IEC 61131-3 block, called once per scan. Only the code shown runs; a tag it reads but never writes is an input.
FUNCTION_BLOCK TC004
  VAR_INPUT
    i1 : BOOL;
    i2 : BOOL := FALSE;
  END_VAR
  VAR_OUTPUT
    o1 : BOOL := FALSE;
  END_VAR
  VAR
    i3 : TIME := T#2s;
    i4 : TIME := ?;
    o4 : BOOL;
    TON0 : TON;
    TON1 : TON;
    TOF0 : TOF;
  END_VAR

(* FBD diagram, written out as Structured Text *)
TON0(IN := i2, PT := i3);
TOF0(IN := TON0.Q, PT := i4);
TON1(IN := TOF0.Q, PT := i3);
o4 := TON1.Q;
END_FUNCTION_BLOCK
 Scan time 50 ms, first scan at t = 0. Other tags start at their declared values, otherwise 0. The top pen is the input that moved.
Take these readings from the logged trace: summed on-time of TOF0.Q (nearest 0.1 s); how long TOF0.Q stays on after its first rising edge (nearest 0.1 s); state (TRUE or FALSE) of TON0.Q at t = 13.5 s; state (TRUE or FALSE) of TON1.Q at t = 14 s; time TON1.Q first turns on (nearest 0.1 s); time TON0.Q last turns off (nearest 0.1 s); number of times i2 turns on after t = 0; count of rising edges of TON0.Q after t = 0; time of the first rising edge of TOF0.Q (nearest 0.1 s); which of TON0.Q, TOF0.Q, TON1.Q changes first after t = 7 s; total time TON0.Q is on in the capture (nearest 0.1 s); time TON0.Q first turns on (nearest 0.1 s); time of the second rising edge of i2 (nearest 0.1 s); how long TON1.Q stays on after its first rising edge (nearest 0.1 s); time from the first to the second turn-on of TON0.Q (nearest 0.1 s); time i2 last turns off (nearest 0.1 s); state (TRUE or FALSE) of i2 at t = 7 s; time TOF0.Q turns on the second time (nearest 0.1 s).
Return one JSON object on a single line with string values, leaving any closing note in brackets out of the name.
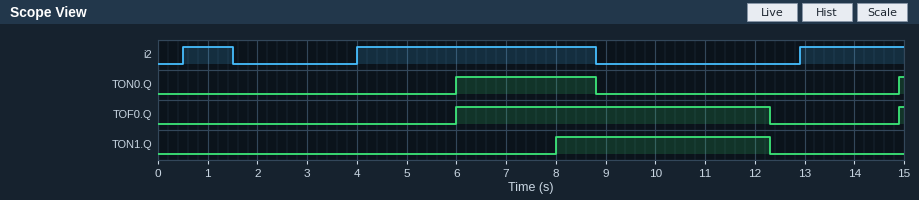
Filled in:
{"summed on-time of TOF0.Q": "6.4 s", "how long TOF0.Q stays on after its first rising edge": "6.3 s", "state (TRUE or FALSE) of TON0.Q at t = 13.5 s": "FALSE", "state (TRUE or FALSE) of TON1.Q at t = 14 s": "FALSE", "time TON1.Q first turns on": "8.0 s", "time TON0.Q last turns off": "8.8 s", "number of times i2 turns on after t = 0": "3", "count of rising edges of TON0.Q after t = 0": "2", "time of the first rising edge of TOF0.Q": "6.0 s", "which of TON0.Q, TOF0.Q, TON1.Q changes first after t = 7 s": "TON1.Q", "total time TON0.Q is on in the capture": "2.9 s", "time TON0.Q first turns on": "6.0 s", "time of the second rising edge of i2": "4.0 s", "how long TON1.Q stays on after its first rising edge": "4.3 s", "time from the first to the second turn-on of TON0.Q": "8.9 s", "time i2 last turns off": "8.8 s", "state (TRUE or FALSE) of i2 at t = 7 s": "TRUE", "time TOF0.Q turns on the second time": "14.9 s"}
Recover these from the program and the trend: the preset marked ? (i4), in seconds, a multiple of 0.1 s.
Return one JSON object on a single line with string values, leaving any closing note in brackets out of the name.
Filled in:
{"the preset marked ? (i4), in seconds, a multiple of 0.1 s": "3.5 s"}
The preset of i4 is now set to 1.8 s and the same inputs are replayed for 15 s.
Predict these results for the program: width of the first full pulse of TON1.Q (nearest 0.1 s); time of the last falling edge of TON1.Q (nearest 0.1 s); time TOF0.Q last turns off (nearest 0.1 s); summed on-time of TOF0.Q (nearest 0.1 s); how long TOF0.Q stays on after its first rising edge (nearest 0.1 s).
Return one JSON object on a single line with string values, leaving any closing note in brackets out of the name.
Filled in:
{"width of the first full pulse of TON1.Q": "2.6 s", "time of the last falling edge of TON1.Q": "10.6 s", "time TOF0.Q last turns off": "10.6 s", "summed on-time of TOF0.Q": "4.7 s", "how long TOF0.Q stays on after its first rising edge": "4.6 s"}
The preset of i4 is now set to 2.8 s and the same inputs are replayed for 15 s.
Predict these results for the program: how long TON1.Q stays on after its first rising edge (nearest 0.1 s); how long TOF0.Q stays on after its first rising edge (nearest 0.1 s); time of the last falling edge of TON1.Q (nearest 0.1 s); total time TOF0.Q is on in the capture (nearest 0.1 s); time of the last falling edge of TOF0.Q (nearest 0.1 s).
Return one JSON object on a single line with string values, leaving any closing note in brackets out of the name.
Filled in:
{"how long TON1.Q stays on after its first rising edge": "3.6 s", "how long TOF0.Q stays on after its first rising edge": "5.6 s", "time of the last falling edge of TON1.Q": "11.6 s", "total time TOF0.Q is on in the capture": "5.7 s", "time of the last falling edge of TOF0.Q": "11.6 s"}
